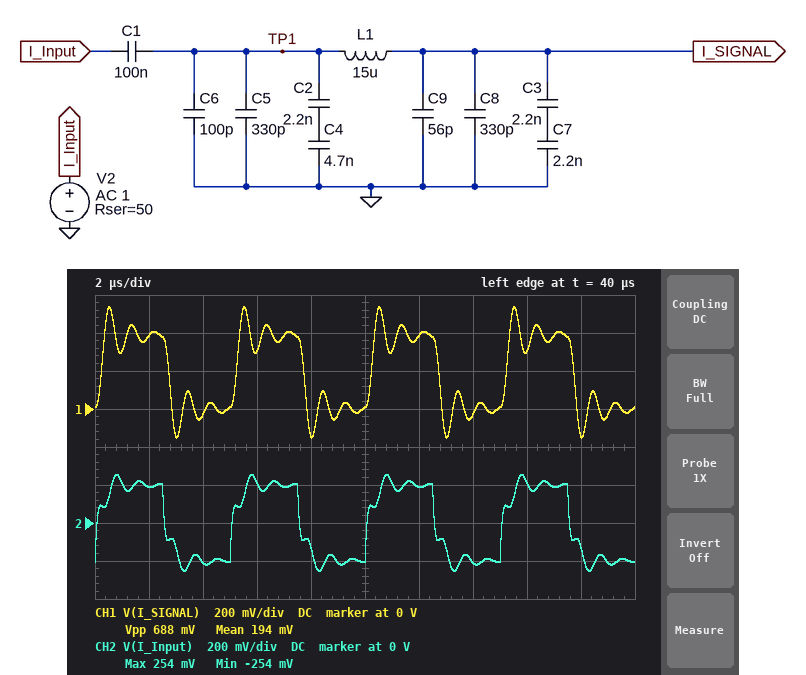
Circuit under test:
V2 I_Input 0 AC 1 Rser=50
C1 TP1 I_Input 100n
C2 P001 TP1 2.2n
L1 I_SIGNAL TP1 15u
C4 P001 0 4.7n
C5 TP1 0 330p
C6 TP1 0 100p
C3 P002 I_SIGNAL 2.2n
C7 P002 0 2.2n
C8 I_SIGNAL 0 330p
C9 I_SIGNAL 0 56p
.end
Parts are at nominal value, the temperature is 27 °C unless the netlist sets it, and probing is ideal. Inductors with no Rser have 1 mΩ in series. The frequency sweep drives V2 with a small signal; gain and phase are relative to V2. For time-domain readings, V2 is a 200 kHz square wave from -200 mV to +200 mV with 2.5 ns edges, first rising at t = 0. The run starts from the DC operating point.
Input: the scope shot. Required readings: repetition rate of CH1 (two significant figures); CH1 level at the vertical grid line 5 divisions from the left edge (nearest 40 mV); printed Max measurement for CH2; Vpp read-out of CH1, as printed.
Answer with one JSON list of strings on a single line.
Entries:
["200 kHz", "0 V", "254 mV", "688 mV"]
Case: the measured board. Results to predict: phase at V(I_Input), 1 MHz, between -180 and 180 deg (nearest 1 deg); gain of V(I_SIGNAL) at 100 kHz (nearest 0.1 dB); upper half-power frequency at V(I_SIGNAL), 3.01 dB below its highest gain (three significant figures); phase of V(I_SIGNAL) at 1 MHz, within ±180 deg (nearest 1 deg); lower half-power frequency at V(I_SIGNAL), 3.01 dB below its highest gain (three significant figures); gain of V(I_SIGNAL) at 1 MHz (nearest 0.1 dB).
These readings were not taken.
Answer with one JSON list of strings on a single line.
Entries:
["-76 deg", "-0.3 dB", "1.36 MHz", "-76 deg", "925 kHz", "5.1 dB"]
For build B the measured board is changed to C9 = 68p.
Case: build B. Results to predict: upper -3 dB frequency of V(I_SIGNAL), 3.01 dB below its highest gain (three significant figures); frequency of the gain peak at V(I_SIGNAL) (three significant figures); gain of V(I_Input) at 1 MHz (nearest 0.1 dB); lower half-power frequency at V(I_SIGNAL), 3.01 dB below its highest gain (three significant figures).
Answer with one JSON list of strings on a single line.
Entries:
["1.35 MHz", "1.17 MHz", "-12.6 dB", "919 kHz"]
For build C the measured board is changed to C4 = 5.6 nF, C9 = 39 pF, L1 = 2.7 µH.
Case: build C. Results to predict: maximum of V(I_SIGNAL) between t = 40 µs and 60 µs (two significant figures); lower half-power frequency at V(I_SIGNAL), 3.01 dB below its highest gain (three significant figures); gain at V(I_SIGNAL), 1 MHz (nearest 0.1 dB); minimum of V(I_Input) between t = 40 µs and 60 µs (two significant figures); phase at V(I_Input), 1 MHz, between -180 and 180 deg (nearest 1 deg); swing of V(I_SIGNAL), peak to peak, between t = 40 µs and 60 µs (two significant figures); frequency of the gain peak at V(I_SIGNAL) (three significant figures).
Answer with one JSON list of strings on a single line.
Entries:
["420 mV", "2.79 MHz", "-2.4 dB", "-220 mV", "-49 deg", "450 mV", "3.17 MHz"]
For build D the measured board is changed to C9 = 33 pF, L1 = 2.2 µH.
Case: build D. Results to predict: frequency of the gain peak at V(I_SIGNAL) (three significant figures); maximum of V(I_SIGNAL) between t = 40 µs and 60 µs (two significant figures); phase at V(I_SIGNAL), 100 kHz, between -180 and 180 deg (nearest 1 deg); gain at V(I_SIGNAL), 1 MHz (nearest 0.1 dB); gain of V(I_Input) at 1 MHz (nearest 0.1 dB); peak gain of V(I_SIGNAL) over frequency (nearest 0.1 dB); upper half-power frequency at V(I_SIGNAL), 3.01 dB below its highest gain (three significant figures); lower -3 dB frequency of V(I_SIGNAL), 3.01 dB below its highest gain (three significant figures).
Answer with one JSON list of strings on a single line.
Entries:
["3.57 MHz", "410 mV", "-6 deg", "-2.5 dB", "-3.4 dB", "3.3 dB", "3.87 MHz", "3.16 MHz"]
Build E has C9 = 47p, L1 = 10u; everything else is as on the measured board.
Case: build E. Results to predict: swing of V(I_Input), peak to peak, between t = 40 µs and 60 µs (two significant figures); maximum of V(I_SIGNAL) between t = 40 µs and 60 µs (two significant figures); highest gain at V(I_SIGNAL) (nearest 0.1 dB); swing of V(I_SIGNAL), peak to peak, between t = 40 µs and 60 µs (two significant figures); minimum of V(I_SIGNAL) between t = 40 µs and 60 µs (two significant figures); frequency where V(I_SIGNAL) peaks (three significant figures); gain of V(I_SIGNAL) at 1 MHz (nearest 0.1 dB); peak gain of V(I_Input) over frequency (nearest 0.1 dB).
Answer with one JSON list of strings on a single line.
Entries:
["500 mV", "510 mV", "5.8 dB", "630 mV", "-120 mV", "1.50 MHz", "1.5 dB", "0 dB"]
